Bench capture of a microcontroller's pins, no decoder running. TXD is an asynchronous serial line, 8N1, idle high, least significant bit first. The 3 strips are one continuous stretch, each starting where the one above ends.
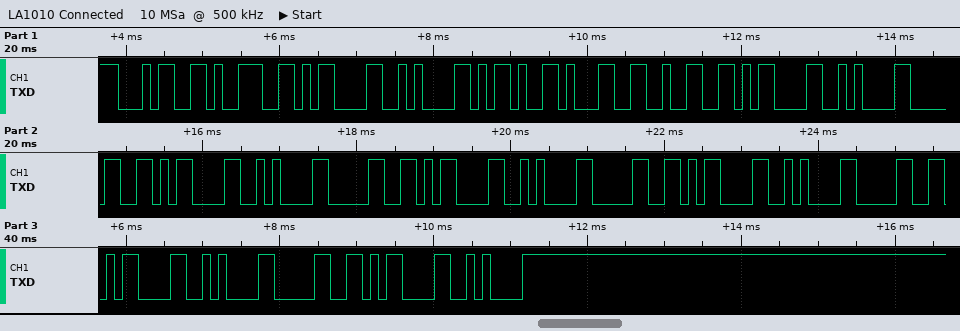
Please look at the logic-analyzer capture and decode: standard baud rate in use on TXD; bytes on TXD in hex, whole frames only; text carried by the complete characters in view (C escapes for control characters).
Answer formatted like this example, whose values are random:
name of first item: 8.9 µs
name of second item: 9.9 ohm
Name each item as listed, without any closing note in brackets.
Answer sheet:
standard baud rate in use on TXD: 9600 baud
bytes on TXD in hex, whole frames only: 0x34 0x39 0x0D 0x0A 0x2D 0x31 0x32 0x0D 0x0A 0x30 0x0D 0x0A 0x30 0x0D 0x0A 0x30 0x0D 0x0A 0x30 0x0D 0x0A 0x30 0x0D 0x0A
text carried by the complete characters in view: "49\r\n-12\r\n0\r\n0\r\n0\r\n0\r\n0\r\n"
